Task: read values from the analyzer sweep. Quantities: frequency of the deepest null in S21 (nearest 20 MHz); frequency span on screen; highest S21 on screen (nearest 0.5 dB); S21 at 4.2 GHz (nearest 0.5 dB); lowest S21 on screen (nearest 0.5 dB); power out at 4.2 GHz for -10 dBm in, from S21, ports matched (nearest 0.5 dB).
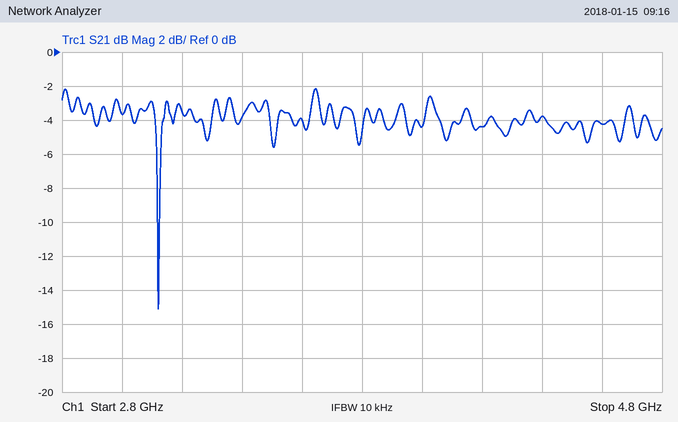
3.12 GHz
2 GHz
-2.0 dB
-4.5 dB
-15.0 dB
-14.5 dBm
